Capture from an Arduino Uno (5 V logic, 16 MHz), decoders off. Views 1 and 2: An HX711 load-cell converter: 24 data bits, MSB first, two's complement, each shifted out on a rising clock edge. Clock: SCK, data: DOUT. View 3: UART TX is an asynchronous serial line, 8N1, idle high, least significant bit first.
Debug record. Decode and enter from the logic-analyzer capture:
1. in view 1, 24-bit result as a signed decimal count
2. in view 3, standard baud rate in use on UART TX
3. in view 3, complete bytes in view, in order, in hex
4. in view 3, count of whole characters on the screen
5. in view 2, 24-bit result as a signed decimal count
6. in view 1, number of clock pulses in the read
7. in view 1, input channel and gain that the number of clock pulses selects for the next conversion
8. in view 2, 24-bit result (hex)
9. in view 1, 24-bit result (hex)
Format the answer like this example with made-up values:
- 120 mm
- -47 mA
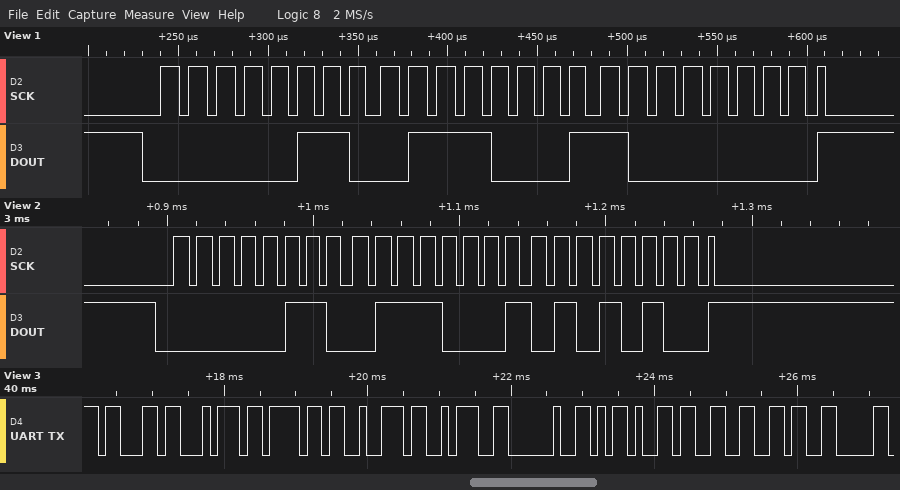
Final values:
- 422272
- 9600 baud
- 63 74 6F 72 3A 20 2D 33 36
- 9
- 422228
- 25
- channel A, gain 128
- 0x067154
- 0x067180
